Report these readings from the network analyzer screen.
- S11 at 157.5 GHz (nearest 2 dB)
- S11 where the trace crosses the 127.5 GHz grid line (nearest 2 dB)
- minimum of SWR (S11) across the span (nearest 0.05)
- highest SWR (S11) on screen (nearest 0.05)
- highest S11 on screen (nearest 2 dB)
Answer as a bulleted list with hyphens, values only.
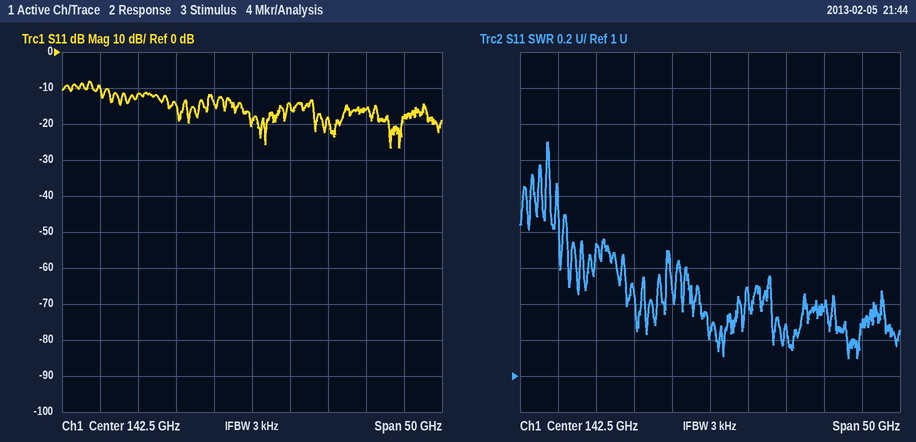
- -16 dB
- -12 dB
- 1.10
- 2.30
- -8 dB
